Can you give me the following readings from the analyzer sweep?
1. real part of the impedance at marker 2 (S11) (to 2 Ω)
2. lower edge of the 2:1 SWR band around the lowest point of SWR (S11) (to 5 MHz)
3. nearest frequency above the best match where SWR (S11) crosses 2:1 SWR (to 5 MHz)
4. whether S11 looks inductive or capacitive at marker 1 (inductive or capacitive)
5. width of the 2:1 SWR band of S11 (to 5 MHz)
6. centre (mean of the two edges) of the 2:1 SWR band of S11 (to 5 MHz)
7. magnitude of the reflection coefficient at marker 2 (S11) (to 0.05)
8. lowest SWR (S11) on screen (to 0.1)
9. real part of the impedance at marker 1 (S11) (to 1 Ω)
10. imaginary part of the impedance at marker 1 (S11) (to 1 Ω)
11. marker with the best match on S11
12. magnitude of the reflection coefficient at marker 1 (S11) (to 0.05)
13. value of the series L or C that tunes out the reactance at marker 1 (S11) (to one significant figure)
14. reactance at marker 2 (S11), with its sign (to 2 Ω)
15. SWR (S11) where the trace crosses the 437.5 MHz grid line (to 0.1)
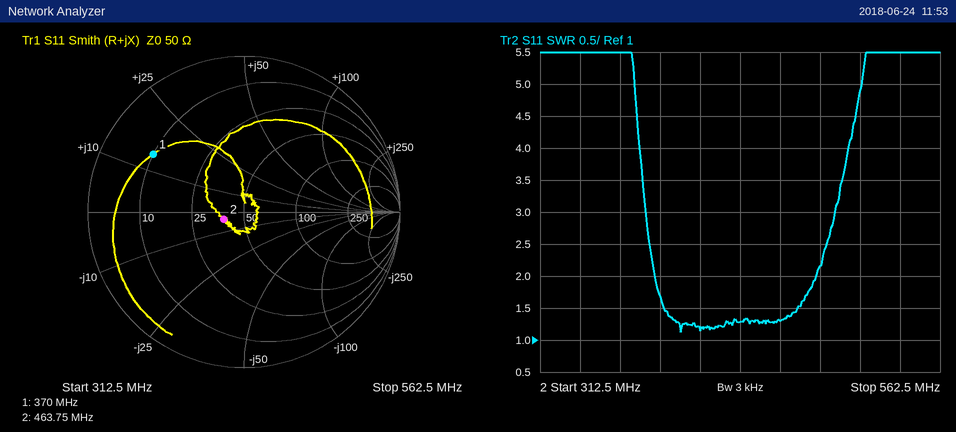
38 Ω
385 MHz
485 MHz
inductive
100 MHz
435 MHz
0.15
1.1
10 Ω
+14 Ω
marker 2
0.70
30 pF
-4 Ω
1.3
